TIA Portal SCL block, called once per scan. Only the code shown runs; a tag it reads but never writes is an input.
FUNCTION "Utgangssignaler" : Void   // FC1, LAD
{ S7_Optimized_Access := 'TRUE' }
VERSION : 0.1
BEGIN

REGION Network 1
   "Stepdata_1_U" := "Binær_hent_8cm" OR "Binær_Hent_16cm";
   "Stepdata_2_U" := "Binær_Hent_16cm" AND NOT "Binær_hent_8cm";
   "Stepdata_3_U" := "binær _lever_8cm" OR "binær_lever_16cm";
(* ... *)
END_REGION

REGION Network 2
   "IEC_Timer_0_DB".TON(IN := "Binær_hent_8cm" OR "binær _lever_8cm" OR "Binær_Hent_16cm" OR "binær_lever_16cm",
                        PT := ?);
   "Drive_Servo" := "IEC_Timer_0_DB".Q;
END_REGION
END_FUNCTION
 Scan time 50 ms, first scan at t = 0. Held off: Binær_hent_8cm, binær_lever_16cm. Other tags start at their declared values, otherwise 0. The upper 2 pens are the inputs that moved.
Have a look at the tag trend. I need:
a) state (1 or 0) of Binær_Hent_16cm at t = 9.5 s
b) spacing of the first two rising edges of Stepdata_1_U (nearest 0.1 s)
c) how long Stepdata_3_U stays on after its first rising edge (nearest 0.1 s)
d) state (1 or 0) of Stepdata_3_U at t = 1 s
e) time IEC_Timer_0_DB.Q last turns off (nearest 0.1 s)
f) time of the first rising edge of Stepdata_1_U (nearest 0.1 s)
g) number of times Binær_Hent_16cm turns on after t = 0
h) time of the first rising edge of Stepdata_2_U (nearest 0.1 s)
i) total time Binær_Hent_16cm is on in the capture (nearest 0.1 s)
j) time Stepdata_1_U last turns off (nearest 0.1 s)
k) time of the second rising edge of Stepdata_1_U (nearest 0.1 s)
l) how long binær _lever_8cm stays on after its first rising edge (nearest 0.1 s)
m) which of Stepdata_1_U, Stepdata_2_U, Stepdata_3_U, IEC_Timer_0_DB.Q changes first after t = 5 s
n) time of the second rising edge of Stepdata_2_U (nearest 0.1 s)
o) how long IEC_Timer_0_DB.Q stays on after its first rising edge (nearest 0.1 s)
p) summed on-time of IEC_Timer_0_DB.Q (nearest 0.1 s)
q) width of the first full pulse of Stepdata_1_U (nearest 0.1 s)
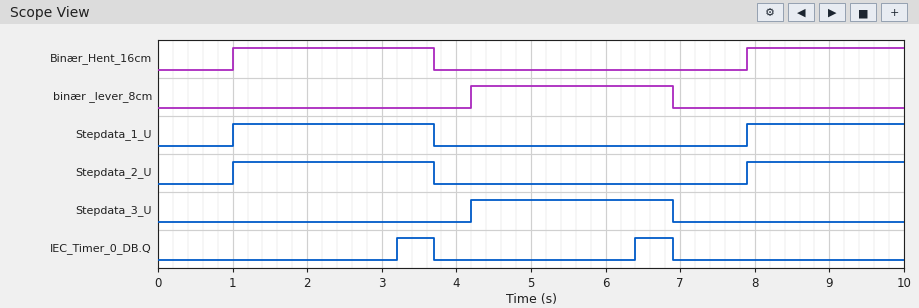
1
6.9 s
2.7 s
0
6.9 s
1.0 s
2
1.0 s
4.8 s
3.7 s
7.9 s
2.7 s
IEC_Timer_0_DB.Q
7.9 s
0.5 s
1.0 s
2.7 s
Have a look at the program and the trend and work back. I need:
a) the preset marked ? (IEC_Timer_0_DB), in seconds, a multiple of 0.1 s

2.2 s
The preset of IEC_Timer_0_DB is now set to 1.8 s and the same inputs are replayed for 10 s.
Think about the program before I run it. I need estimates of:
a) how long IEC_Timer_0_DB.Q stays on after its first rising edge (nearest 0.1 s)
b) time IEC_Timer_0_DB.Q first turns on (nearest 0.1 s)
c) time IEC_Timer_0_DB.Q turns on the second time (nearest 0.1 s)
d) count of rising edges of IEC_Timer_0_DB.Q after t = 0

0.9 s
2.8 s
6.0 s
3
